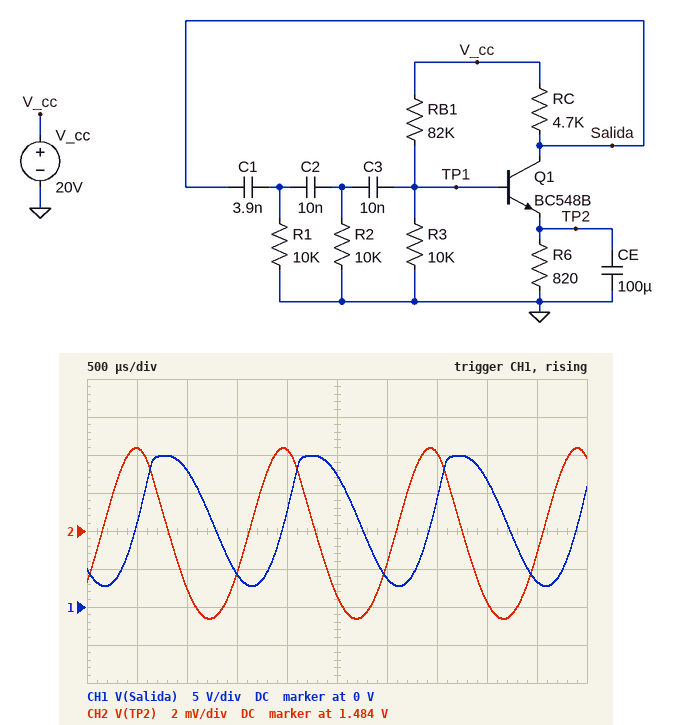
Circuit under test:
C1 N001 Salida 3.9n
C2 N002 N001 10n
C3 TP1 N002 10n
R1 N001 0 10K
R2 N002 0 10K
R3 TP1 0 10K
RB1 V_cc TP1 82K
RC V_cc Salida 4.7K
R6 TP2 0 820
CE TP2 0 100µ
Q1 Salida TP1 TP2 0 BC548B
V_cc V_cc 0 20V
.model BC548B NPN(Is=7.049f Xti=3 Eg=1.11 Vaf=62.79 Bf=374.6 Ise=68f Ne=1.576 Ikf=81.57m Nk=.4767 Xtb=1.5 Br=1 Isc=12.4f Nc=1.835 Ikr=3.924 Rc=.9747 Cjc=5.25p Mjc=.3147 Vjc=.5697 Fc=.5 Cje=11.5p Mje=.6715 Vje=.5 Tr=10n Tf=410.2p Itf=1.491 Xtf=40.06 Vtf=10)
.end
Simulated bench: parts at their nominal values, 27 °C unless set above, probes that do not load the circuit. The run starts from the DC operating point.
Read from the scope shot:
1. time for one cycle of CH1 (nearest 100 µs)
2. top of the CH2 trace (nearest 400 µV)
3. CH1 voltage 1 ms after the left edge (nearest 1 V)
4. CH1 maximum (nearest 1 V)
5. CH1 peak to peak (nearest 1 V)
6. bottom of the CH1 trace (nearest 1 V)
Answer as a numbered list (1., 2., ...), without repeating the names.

1. 1.5 ms
2. 1.4884 V
3. 18 V
4. 20 V
5. 17 V
6. 3 V
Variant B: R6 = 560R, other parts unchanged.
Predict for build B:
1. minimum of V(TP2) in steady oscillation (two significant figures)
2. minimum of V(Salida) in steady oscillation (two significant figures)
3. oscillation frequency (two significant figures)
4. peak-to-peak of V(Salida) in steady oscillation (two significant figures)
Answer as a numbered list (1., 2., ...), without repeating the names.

1. 1.4 V
2. 1.5 V
3. 710 Hz
4. 14 V
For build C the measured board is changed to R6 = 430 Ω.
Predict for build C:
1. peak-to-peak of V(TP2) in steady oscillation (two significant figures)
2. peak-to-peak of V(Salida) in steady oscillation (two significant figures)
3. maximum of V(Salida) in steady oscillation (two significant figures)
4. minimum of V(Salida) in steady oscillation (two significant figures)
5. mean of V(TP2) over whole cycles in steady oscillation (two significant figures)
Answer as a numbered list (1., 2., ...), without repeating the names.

1. 3.6 mV
2. 7.2 V
3. 8.7 V
4. 1.5 V
5. 1.4 V
